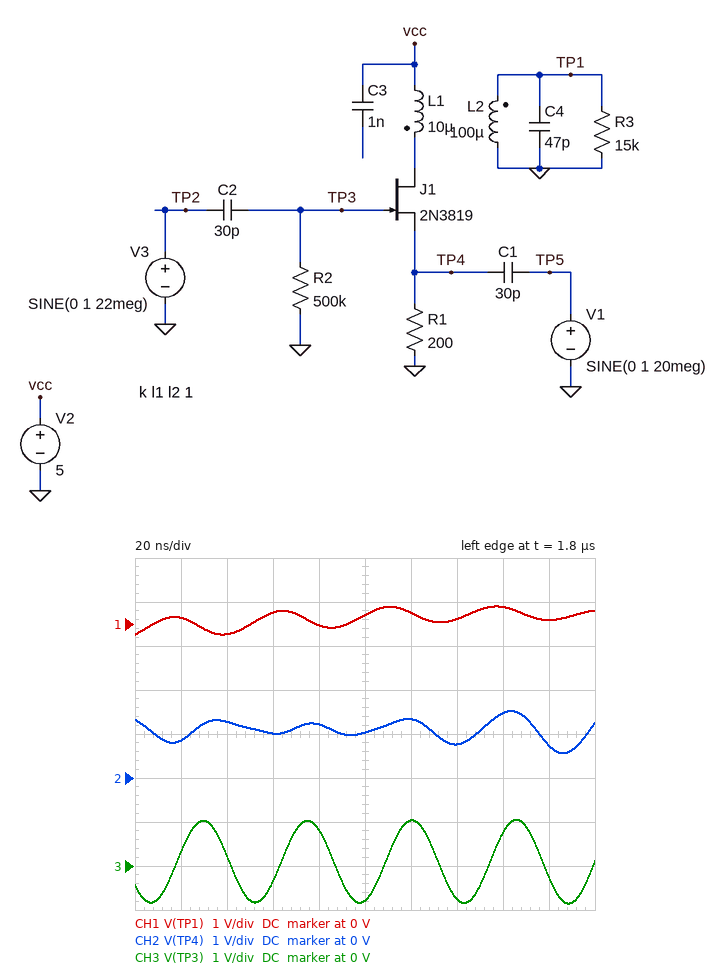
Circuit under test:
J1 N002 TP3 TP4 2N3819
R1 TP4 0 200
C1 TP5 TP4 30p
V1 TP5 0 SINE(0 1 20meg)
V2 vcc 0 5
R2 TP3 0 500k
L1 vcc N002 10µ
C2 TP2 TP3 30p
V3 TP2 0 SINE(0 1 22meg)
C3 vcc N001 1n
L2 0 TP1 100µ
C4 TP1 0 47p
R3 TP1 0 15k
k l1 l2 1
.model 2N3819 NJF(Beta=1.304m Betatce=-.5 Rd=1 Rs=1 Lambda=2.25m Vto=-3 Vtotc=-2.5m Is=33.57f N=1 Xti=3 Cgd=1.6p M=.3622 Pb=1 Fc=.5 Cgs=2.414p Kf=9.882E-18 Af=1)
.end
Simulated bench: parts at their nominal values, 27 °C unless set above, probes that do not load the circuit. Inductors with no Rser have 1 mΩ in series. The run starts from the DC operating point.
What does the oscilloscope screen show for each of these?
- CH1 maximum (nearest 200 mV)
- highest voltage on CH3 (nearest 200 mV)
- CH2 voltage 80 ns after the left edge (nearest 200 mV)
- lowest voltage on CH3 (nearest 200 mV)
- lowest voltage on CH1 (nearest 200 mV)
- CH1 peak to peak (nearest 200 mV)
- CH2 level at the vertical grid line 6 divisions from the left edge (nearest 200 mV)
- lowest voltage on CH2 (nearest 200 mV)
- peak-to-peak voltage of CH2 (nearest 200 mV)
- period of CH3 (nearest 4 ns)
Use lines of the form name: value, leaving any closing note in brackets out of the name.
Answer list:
CH1 maximum: 400 mV
highest voltage on CH3: 1.0 V
CH2 voltage 80 ns after the left edge: 1.2 V
lowest voltage on CH3: -800 mV
lowest voltage on CH1: -200 mV
CH1 peak to peak: 600 mV
CH2 level at the vertical grid line 6 divisions from the left edge: 1.4 V
lowest voltage on CH2: 600 mV
peak-to-peak voltage of CH2: 1.0 V
period of CH3: 44 ns
